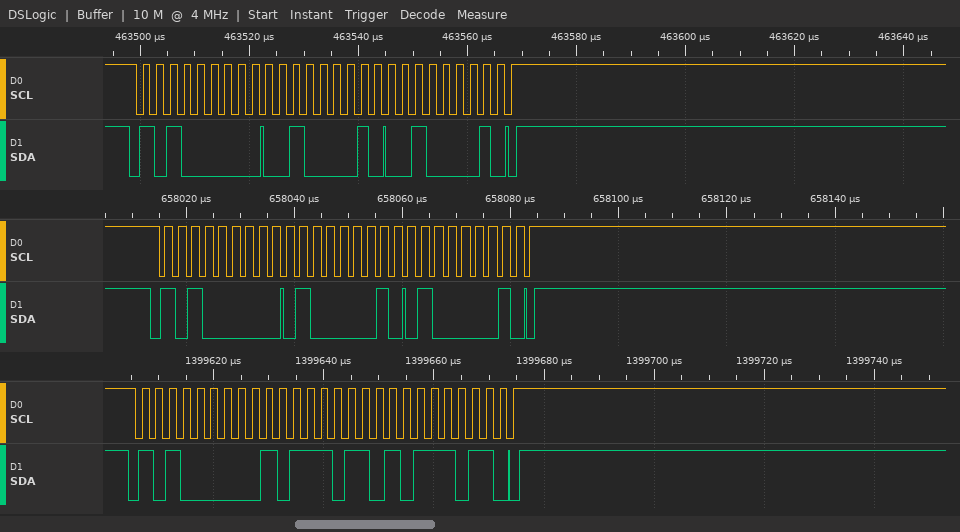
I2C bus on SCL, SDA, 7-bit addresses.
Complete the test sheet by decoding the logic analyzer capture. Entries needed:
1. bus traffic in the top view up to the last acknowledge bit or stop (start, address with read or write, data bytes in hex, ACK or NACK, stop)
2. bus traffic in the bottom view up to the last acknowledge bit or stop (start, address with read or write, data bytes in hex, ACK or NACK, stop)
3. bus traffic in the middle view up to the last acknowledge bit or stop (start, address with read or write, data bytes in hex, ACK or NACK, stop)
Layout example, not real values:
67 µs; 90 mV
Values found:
start, address 50 write ACK, 21 ACK, 21 ACK, stop; start, address 50 write ACK, BB ACK, BB ACK, stop; start, address 50 write ACK, 41 ACK, 41 ACK, stop
